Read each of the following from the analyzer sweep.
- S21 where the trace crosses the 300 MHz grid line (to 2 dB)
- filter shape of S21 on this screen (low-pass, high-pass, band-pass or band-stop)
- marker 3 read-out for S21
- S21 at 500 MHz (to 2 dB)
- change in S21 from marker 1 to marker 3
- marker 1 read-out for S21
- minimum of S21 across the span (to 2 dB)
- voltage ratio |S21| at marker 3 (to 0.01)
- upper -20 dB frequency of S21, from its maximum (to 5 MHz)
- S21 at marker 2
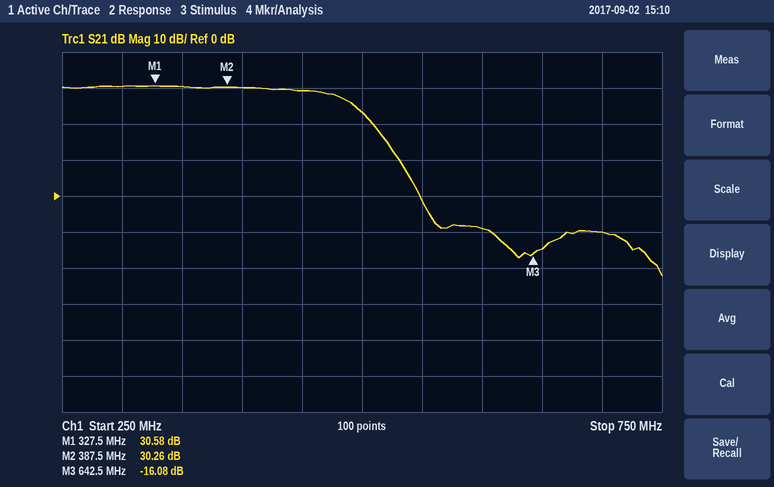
30 dB
low-pass
-16.08 dB
24 dB
-46.66 dB
30.58 dB
-22 dB
0.16
530 MHz
30.26 dB
